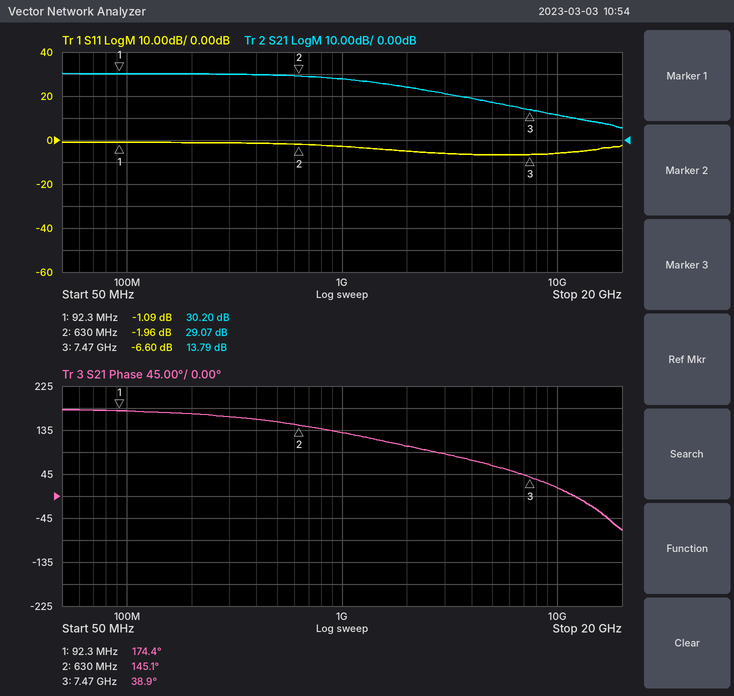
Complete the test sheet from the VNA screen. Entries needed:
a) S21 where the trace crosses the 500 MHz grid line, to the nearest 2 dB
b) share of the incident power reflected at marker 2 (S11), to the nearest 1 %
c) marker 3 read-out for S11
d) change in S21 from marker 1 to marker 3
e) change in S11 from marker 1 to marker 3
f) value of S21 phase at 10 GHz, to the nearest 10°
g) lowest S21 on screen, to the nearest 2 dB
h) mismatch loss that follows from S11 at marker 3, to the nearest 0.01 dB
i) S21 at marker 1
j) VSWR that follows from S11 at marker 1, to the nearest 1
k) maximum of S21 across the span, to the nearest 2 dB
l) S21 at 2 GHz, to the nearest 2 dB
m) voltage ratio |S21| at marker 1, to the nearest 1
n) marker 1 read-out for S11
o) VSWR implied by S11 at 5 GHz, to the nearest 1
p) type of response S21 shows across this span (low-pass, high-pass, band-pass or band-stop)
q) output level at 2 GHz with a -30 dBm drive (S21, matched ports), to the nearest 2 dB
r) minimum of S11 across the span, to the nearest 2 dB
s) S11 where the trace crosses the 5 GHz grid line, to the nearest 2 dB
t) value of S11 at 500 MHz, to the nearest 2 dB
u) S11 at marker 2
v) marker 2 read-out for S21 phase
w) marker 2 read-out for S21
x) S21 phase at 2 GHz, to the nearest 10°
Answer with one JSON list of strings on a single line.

["30 dB", "64 %", "-6.60 dB", "-16.41 dB", "-5.51 dB", "20°", "6 dB", "1.07 dB", "30.20 dB", "16", "30 dB", "24 dB", "32", "-1.09 dB", "3", "low-pass", "-6 dBm", "-6 dB", "-6 dB", "-2 dB", "-1.96 dB", "145.1°", "29.07 dB", "100°"]
